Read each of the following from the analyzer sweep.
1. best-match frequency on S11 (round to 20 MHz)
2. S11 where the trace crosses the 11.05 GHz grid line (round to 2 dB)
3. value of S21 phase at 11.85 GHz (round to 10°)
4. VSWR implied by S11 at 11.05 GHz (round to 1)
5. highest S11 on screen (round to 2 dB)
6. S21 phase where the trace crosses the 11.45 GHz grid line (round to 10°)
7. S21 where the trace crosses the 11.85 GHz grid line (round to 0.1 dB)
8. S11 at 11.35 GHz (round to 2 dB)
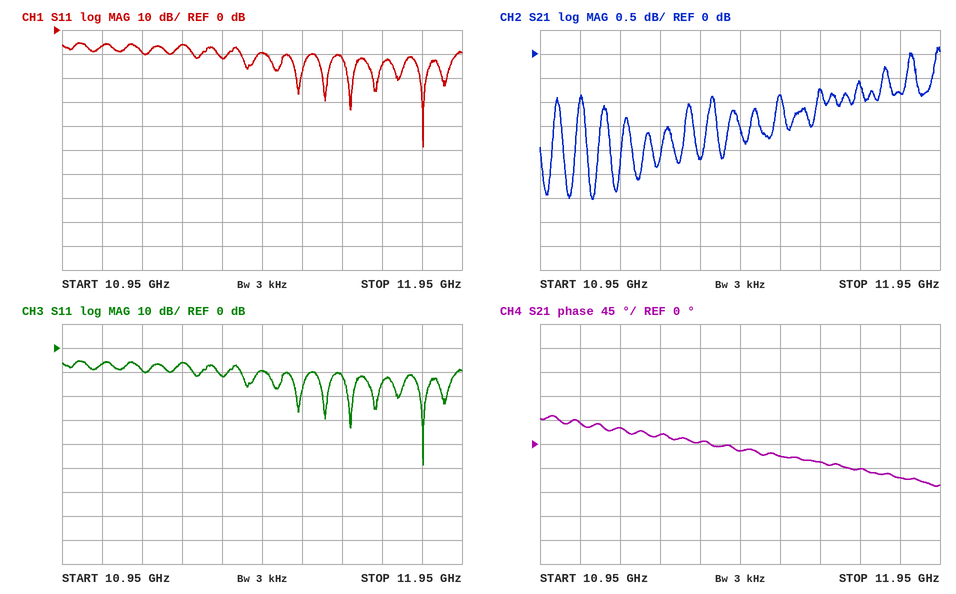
11.86 GHz
-6 dB
-60°
3
-6 dB
-10°
-0.8 dB
-12 dB
